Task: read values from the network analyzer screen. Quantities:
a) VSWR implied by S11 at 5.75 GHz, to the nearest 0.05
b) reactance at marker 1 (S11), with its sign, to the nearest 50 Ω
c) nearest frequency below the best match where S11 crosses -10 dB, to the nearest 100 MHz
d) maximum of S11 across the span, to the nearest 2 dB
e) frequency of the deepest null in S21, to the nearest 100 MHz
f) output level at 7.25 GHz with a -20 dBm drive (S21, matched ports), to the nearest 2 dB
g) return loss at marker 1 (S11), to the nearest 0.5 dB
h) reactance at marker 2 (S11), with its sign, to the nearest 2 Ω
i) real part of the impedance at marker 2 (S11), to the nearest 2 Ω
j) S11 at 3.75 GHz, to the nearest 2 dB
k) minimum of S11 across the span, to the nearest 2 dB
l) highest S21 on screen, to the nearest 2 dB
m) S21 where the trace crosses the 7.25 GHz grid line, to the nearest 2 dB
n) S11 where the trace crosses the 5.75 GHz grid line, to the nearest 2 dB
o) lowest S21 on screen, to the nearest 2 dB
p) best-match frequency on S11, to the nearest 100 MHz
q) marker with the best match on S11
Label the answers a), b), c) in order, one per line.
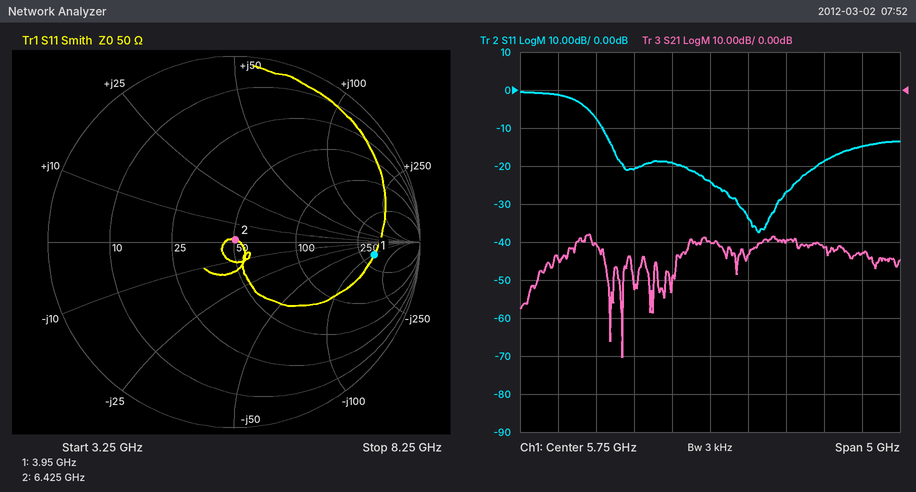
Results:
a) 1.15
b) -100 Ω
c) 4.3 GHz
d) 0 dB
e) 4.6 GHz
f) -62 dBm
g) 2.5 dB
h) +2 Ω
i) 50 Ω
j) -2 dB
k) -38 dB
l) -38 dB
m) -42 dB
n) -24 dB
o) -70 dB
p) 6.4 GHz
q) marker 2
